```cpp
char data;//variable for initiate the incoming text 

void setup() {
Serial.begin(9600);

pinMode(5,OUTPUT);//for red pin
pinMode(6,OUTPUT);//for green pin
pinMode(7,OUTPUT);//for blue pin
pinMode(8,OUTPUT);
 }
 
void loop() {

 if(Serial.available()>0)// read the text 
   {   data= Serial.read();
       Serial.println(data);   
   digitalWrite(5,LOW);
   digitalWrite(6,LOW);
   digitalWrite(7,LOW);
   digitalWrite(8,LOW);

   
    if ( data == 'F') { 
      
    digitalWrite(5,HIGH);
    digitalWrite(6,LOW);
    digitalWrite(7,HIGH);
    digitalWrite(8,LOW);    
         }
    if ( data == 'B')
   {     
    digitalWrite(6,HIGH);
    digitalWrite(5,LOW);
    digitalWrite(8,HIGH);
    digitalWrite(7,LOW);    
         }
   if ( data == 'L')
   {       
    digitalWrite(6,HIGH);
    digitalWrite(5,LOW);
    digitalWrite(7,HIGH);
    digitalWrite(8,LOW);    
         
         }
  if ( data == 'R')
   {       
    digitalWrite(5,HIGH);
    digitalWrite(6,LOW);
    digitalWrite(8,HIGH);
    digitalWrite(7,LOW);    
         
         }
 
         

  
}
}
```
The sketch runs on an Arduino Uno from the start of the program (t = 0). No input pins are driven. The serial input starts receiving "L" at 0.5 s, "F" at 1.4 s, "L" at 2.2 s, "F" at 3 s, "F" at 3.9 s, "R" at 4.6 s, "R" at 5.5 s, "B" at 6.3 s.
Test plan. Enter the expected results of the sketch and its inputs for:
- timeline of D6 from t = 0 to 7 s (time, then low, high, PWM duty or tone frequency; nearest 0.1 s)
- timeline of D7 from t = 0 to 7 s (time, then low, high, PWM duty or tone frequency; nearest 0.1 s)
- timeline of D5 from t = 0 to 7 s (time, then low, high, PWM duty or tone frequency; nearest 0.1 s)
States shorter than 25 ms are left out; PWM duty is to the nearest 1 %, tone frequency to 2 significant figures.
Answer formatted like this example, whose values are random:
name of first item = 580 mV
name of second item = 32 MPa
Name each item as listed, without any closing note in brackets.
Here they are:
timeline of D6 from t = 0 to 7 s = 0 s low; 0.5 s high; 1.4 s low; 2.2 s high; 3 s low; 6.3 s high
timeline of D7 from t = 0 to 7 s = 0 s low; 0.5 s high; 4.6 s low
timeline of D5 from t = 0 to 7 s = 0 s low; 1.4 s high; 2.2 s low; 3 s high; 6.3 s low
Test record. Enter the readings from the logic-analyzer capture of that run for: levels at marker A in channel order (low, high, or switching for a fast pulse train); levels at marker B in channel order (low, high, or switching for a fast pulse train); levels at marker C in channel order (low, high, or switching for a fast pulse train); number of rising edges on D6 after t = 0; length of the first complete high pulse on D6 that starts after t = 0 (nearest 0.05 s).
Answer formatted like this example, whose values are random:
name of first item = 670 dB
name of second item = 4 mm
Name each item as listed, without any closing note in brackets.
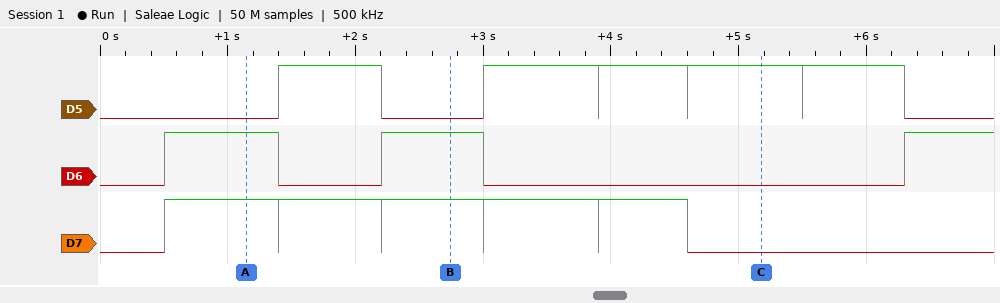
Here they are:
levels at marker A in channel order = D5 low, D6 high, D7 high
levels at marker B in channel order = D5 low, D6 high, D7 high
levels at marker C in channel order = D5 high, D6 low, D7 low
number of rising edges on D6 after t = 0 = 3
length of the first complete high pulse on D6 that starts after t = 0 = 0.90 s
